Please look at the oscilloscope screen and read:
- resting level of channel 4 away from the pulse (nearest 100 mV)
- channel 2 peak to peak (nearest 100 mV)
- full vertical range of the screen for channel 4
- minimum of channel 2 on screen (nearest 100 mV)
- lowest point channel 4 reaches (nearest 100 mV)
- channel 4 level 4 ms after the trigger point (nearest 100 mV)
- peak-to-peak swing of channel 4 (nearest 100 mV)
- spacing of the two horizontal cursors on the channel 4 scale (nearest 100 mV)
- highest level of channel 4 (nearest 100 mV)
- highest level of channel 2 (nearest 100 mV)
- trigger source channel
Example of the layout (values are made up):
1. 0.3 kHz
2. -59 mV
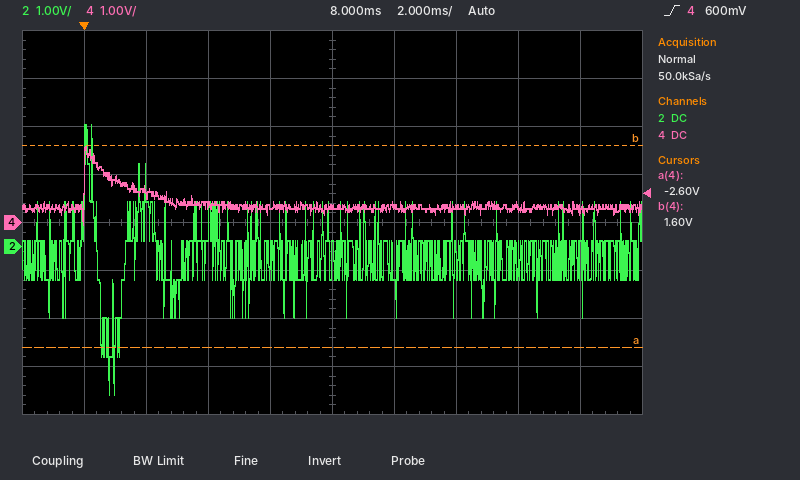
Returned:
1. 300 mV
2. 5.6 V
3. 8 V
4. -3.1 V
5. 0.0 V
6. 400 mV
7. 1.6 V
8. 4.2 V
9. 1.6 V
10. 2.5 V
11. channel 4
